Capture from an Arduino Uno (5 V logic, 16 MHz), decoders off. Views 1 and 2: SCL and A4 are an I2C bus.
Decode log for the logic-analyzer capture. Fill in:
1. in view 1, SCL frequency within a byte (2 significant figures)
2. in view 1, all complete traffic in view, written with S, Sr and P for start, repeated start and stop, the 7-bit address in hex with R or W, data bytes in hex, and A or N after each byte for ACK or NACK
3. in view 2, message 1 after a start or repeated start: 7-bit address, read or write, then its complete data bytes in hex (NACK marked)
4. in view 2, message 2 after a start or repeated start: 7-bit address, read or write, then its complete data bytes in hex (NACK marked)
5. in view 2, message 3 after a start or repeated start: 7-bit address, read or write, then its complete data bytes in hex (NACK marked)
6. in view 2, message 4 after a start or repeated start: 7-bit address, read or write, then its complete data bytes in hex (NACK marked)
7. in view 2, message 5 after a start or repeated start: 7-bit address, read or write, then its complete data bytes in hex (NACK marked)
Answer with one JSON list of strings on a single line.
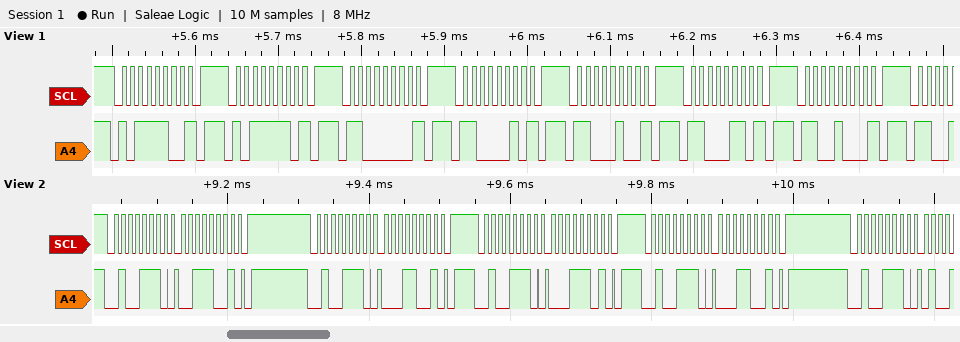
["100 kHz", "S 5EW N P S 5FW N P S 60W N P S 61W N P S 62W N P S 63W N P S 64W N P", "0x27 write: 39", "0x27 write: 19", "0x27 write: 1D", "0x27 write: 19", "0x27 write"]
